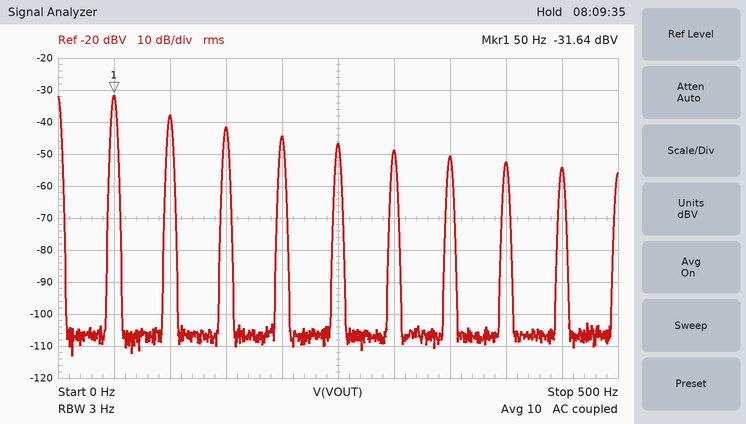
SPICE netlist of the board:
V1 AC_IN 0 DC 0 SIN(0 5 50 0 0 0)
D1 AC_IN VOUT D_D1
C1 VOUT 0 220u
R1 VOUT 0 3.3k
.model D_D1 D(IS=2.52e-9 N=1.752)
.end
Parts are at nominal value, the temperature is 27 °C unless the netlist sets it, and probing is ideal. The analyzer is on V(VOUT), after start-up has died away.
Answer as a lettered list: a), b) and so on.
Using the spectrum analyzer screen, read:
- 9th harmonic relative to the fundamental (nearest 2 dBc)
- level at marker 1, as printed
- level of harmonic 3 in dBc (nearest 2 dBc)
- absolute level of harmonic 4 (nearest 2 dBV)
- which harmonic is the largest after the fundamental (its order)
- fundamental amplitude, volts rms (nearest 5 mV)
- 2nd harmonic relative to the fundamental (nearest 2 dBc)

a) -22 dBc
b) -31.64 dBV
c) -10 dBc
d) -44 dBV
e) 2
f) 25 mV
g) -6 dBc
